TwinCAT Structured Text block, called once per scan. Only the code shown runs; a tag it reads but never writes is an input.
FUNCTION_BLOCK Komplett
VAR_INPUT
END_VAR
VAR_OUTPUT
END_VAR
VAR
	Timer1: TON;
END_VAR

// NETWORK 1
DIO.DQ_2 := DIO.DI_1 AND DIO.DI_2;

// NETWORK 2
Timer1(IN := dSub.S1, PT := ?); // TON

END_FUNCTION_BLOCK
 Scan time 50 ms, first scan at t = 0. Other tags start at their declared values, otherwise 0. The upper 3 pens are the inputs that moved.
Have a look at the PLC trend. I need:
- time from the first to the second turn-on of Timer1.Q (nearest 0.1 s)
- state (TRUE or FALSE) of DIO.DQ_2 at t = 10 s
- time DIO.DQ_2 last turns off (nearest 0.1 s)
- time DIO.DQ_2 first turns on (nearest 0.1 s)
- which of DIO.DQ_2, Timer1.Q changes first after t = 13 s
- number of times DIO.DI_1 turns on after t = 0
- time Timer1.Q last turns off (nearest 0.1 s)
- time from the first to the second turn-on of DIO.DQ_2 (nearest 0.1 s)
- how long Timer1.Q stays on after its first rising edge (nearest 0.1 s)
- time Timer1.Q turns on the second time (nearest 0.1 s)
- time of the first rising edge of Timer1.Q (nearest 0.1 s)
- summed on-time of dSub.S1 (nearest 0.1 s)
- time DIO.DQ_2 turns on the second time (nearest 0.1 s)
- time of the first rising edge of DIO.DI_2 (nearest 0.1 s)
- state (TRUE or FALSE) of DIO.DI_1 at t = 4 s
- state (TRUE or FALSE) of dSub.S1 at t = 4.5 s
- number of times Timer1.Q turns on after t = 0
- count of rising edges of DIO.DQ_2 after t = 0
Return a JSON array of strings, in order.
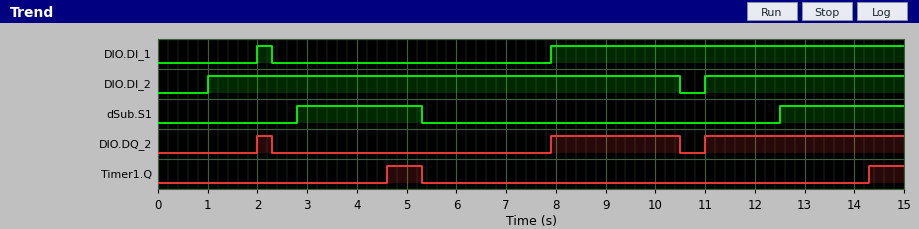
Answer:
["9.7 s", "TRUE", "10.5 s", "2.0 s", "Timer1.Q", "2", "5.3 s", "5.9 s", "0.7 s", "14.3 s", "4.6 s", "5.0 s", "7.9 s", "1.0 s", "FALSE", "TRUE", "2", "3"]
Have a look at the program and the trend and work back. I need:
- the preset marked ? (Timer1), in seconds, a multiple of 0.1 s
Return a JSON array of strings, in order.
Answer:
["1.8 s"]
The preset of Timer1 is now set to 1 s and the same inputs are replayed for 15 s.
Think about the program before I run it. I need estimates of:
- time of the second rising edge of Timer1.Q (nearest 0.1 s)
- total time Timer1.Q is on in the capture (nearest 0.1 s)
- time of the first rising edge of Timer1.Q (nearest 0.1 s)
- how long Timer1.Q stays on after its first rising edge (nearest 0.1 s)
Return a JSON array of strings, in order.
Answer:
["13.5 s", "3.0 s", "3.8 s", "1.5 s"]
